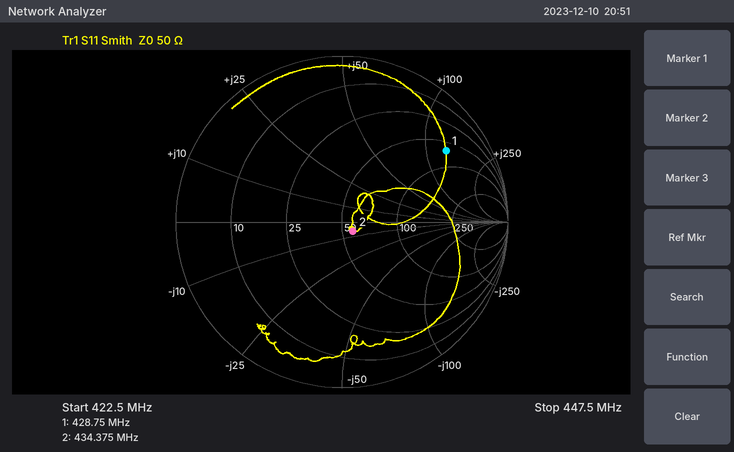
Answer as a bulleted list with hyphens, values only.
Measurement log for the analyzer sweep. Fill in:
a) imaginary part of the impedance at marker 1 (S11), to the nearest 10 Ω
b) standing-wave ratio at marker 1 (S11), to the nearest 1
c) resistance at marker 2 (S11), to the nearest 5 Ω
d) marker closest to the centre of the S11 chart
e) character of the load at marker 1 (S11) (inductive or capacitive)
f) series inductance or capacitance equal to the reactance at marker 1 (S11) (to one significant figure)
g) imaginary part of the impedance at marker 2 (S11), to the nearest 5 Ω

- +130 Ω
- 7
- 55 Ω
- marker 2
- inductive
- 50 nH
- -5 Ω
